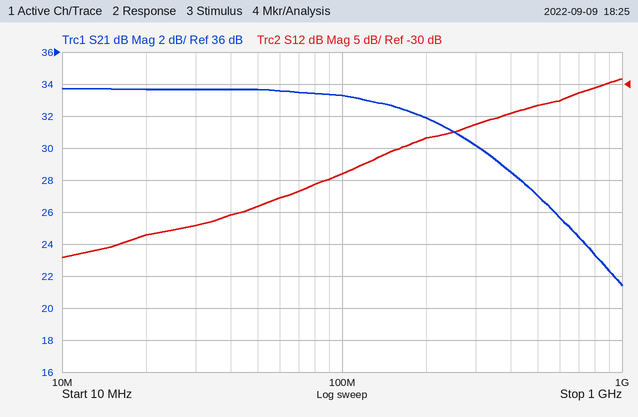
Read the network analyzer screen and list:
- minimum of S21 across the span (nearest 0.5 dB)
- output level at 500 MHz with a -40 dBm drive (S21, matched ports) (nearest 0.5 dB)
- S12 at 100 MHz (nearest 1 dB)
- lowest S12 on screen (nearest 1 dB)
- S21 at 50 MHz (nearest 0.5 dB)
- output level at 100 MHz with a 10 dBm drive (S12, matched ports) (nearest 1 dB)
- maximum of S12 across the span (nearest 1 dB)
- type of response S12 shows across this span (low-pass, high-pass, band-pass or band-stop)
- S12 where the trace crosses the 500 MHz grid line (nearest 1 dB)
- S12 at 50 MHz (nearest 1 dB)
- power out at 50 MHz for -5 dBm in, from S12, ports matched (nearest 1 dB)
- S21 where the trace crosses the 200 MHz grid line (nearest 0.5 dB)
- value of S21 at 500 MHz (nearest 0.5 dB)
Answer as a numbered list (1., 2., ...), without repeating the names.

1. 21.5 dB
2. -13.0 dBm
3. -44 dB
4. -57 dB
5. 33.5 dB
6. -34 dBm
7. -29 dB
8. high-pass
9. -33 dB
10. -49 dB
11. -54 dBm
12. 32.0 dB
13. 27.0 dB
